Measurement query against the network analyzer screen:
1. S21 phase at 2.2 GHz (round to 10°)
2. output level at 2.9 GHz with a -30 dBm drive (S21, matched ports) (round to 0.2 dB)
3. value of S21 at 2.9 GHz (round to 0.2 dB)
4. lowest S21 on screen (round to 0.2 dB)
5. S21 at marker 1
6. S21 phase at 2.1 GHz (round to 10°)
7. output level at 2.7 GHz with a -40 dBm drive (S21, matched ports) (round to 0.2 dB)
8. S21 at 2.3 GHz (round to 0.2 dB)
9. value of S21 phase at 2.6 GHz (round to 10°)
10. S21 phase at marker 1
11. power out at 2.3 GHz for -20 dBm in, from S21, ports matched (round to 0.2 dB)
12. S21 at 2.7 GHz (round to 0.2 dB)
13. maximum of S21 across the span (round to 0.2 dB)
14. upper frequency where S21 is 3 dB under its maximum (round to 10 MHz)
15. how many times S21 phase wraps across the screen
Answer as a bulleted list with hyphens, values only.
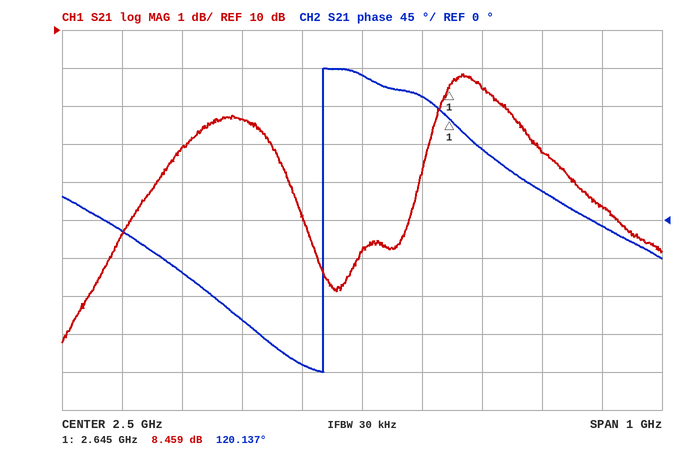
- -60°
- -24.6 dBm
- 5.4 dB
- 1.8 dB
- 8.459 dB
- -10°
- -31.6 dBm
- 7.6 dB
- 150°
- 120.137°
- -12.4 dBm
- 8.4 dB
- 8.8 dB
- 2.86 GHz
- 1
